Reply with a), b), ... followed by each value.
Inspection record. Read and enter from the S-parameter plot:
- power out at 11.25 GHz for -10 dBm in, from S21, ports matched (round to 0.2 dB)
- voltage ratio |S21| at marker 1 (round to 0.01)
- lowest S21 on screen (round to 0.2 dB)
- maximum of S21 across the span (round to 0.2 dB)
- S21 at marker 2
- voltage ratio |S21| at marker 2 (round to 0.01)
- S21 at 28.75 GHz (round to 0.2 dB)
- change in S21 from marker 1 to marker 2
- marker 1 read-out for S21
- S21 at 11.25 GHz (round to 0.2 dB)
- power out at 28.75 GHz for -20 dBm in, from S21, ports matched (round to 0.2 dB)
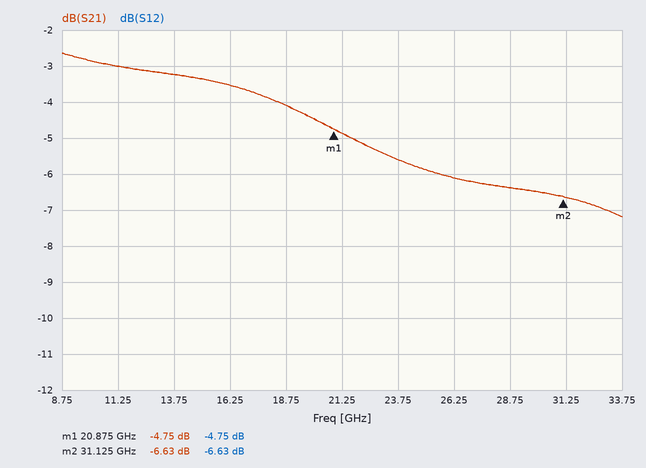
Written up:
a) -13.0 dBm
b) 0.58
c) -7.2 dB
d) -2.6 dB
e) -6.63 dB
f) 0.47
g) -6.4 dB
h) -1.88 dB
i) -4.75 dB
j) -3.0 dB
k) -26.4 dBm
